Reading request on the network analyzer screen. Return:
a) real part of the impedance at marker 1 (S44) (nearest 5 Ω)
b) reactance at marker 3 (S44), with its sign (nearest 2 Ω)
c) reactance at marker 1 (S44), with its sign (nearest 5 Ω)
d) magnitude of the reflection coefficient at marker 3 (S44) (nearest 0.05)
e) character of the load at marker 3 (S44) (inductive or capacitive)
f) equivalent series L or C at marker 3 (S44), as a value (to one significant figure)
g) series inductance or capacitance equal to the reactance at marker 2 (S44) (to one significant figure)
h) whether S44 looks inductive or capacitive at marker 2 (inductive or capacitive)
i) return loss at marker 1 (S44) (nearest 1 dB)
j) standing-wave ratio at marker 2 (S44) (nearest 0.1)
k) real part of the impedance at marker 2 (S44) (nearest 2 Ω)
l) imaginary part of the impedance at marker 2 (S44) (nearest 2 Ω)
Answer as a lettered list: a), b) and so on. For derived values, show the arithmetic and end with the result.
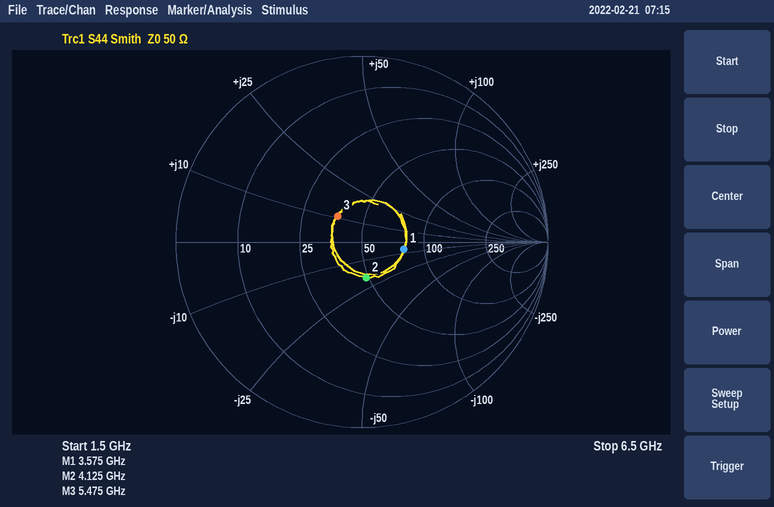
a) 80 Ω
b) +10 Ω
c) -5 Ω
d) 0.20
e) inductive
f) L = 10 Ω/(2π × 5.475 GHz) ≈ 291 pH, so 300 pH to one significant figure
g) C = 1/(2π × 4.125 GHz × 20 Ω) ≈ 2 pF
h) capacitive
i) 13 dB
j) 1.5
k) 48 Ω
l) -20 Ω
